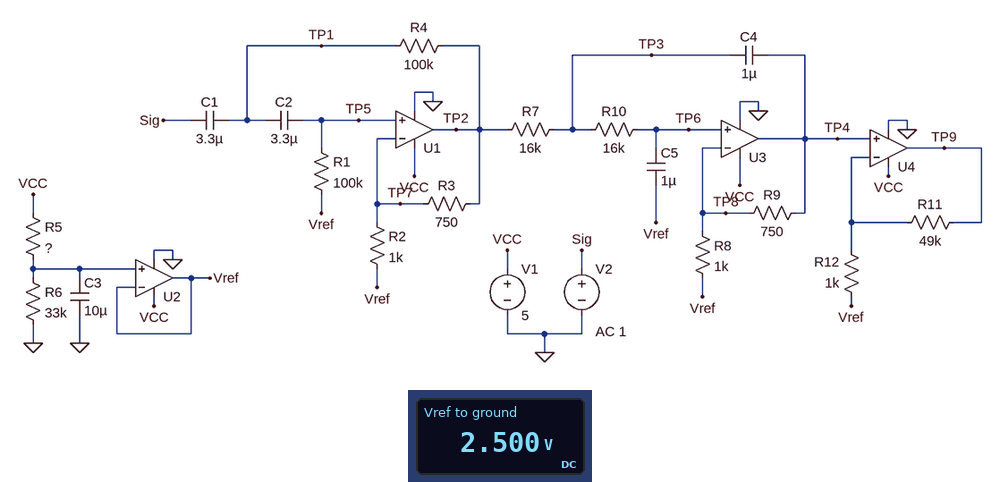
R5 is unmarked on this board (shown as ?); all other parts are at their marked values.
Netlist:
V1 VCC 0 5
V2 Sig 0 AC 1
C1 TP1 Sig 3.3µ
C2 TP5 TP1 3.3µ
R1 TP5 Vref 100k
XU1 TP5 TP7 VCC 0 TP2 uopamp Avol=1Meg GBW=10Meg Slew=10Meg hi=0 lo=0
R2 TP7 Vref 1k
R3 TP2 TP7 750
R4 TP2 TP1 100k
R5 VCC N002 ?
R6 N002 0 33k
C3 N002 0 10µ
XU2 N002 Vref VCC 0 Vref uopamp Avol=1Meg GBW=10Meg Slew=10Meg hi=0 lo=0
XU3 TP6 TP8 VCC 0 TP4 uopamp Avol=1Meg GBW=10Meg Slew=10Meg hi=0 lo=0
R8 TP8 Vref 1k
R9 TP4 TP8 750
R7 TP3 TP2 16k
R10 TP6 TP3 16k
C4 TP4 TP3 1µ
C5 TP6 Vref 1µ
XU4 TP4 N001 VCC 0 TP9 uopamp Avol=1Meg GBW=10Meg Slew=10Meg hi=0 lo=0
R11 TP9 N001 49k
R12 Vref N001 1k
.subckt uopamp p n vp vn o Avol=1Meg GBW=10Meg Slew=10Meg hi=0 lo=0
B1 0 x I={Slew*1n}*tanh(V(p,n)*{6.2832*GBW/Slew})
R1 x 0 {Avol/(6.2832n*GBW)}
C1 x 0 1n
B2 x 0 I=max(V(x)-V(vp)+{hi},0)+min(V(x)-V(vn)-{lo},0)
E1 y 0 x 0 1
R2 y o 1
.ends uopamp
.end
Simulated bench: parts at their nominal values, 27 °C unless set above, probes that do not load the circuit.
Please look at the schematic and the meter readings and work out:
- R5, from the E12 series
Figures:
33 kΩ
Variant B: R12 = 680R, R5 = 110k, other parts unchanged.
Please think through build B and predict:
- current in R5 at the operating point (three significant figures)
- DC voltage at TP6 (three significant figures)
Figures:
35.0 µA
1.15 V
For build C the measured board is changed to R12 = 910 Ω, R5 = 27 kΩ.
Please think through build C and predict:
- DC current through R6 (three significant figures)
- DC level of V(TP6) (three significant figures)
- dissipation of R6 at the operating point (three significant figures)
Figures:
83.3 µA
2.75 V
229 µW
